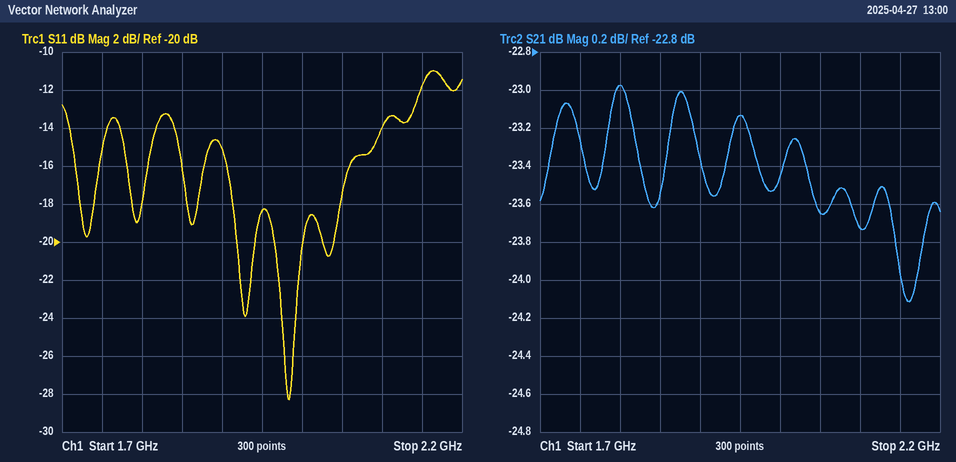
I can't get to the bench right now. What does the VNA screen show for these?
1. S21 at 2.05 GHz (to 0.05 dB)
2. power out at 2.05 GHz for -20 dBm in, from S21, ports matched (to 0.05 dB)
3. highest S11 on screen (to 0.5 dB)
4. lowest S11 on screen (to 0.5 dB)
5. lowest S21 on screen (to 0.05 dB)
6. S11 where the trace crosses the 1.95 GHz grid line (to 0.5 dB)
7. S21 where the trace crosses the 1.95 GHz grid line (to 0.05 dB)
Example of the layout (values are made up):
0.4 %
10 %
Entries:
-23.65 dB
-43.65 dBm
-11.0 dB
-28.5 dB
-24.10 dB
-18.5 dB
-23.15 dB
